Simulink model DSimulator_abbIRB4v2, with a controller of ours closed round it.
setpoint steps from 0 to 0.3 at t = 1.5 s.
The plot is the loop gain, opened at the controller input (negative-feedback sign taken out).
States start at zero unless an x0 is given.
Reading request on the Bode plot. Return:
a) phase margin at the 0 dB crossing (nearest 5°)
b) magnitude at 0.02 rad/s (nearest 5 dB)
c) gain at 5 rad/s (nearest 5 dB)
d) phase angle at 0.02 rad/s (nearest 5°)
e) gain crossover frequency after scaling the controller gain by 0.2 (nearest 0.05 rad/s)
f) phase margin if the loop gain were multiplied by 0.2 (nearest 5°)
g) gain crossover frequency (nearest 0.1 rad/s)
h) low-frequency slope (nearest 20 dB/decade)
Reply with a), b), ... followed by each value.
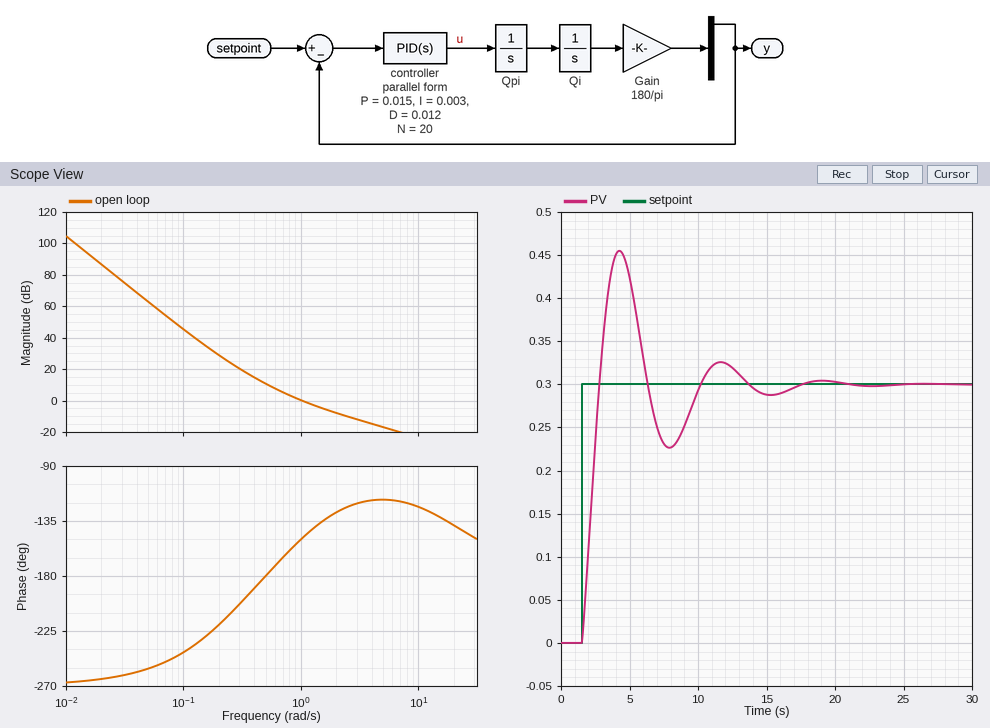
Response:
a) 30°
b) 85 dB
c) -15 dB
d) -265°
e) 0.40 rad/s
f) -10°
g) 1.0 rad/s
h) -60 dB/decade
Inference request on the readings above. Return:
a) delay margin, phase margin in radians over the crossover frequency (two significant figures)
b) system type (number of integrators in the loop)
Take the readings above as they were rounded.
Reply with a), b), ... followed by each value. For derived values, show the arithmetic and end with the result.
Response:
a) 30 × π / 180 / 1 = 0.52 s
b) 3
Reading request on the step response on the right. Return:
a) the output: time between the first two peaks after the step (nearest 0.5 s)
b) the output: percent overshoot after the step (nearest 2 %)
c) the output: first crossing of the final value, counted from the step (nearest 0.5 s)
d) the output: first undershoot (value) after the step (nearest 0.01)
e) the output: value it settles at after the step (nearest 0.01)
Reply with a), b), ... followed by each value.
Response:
a) 7.5 s
b) 52 %
c) 1.5 s
d) 0.23
e) 0.30
